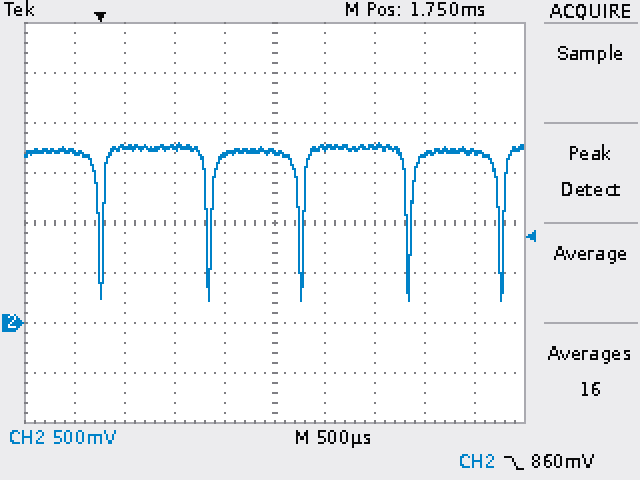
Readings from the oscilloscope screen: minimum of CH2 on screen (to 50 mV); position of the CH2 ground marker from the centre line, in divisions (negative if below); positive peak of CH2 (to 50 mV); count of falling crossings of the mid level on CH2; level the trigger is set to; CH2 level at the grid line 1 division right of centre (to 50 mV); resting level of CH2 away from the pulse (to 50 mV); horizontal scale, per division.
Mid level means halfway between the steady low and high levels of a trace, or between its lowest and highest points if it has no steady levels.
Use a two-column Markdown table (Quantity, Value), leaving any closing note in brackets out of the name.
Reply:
| Quantity | Value |
|---|---|
| minimum of CH2 on screen | 200 mV |
| position of the CH2 ground marker from the centre line, in divisions | -2.0 div |
| positive peak of CH2 | 1.80 V |
| count of falling crossings of the mid level on CH2 | 5 |
| level the trigger is set to | 860 mV |
| CH2 level at the grid line 1 division right of centre | 1.75 V |
| resting level of CH2 away from the pulse | 1.75 V |
| horizontal scale, per division | 500 µs |
